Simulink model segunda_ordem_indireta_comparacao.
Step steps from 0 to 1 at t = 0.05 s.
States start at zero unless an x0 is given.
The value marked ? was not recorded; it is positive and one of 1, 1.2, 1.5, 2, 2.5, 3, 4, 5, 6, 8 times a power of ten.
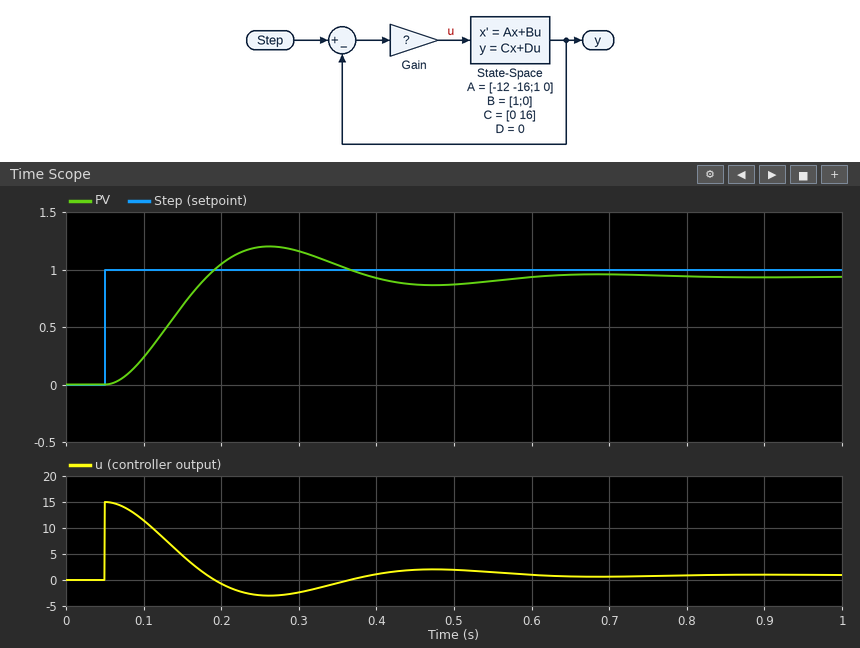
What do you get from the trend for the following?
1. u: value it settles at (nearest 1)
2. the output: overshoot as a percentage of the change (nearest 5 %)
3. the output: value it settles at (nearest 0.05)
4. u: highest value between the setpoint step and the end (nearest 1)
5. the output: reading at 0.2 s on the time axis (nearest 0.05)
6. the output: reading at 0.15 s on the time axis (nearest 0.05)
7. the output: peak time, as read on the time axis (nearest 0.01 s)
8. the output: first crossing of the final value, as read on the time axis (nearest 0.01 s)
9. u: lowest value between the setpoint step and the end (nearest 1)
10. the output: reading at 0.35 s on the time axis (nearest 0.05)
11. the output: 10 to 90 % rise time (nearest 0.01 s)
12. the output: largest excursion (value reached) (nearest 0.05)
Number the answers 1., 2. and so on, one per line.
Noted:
1. 1
2. 30 %
3. 0.95
4. 15
5. 1.05
6. 0.70
7. 0.26 s
8. 0.18 s
9. -3
10. 1.05
11. 0.09 s
12. 1.20
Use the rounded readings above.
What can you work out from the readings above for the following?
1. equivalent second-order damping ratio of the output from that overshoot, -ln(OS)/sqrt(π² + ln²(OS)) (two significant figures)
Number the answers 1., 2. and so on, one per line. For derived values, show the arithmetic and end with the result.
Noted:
1. ln(0.3) = -1.204; 1.204 / sqrt(9.870 + 1.450) = 0.36
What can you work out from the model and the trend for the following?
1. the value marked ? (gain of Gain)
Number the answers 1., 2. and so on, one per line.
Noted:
1. 15
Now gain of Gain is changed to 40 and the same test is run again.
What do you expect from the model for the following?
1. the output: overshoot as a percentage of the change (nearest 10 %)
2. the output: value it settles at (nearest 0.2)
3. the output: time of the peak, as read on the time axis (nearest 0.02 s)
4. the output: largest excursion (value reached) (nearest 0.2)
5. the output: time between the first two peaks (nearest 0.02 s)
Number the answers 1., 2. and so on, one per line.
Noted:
1. 50 %
2. 1.0
3. 0.18 s
4. 1.4
5. 0.26 s
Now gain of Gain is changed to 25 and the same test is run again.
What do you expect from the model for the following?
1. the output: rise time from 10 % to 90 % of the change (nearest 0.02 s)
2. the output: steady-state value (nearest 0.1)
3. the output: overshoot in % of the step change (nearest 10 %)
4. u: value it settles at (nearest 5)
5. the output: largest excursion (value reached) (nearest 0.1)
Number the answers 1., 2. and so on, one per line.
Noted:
1. 0.06 s
2. 1.0
3. 40 %
4. 0
5. 1.3
